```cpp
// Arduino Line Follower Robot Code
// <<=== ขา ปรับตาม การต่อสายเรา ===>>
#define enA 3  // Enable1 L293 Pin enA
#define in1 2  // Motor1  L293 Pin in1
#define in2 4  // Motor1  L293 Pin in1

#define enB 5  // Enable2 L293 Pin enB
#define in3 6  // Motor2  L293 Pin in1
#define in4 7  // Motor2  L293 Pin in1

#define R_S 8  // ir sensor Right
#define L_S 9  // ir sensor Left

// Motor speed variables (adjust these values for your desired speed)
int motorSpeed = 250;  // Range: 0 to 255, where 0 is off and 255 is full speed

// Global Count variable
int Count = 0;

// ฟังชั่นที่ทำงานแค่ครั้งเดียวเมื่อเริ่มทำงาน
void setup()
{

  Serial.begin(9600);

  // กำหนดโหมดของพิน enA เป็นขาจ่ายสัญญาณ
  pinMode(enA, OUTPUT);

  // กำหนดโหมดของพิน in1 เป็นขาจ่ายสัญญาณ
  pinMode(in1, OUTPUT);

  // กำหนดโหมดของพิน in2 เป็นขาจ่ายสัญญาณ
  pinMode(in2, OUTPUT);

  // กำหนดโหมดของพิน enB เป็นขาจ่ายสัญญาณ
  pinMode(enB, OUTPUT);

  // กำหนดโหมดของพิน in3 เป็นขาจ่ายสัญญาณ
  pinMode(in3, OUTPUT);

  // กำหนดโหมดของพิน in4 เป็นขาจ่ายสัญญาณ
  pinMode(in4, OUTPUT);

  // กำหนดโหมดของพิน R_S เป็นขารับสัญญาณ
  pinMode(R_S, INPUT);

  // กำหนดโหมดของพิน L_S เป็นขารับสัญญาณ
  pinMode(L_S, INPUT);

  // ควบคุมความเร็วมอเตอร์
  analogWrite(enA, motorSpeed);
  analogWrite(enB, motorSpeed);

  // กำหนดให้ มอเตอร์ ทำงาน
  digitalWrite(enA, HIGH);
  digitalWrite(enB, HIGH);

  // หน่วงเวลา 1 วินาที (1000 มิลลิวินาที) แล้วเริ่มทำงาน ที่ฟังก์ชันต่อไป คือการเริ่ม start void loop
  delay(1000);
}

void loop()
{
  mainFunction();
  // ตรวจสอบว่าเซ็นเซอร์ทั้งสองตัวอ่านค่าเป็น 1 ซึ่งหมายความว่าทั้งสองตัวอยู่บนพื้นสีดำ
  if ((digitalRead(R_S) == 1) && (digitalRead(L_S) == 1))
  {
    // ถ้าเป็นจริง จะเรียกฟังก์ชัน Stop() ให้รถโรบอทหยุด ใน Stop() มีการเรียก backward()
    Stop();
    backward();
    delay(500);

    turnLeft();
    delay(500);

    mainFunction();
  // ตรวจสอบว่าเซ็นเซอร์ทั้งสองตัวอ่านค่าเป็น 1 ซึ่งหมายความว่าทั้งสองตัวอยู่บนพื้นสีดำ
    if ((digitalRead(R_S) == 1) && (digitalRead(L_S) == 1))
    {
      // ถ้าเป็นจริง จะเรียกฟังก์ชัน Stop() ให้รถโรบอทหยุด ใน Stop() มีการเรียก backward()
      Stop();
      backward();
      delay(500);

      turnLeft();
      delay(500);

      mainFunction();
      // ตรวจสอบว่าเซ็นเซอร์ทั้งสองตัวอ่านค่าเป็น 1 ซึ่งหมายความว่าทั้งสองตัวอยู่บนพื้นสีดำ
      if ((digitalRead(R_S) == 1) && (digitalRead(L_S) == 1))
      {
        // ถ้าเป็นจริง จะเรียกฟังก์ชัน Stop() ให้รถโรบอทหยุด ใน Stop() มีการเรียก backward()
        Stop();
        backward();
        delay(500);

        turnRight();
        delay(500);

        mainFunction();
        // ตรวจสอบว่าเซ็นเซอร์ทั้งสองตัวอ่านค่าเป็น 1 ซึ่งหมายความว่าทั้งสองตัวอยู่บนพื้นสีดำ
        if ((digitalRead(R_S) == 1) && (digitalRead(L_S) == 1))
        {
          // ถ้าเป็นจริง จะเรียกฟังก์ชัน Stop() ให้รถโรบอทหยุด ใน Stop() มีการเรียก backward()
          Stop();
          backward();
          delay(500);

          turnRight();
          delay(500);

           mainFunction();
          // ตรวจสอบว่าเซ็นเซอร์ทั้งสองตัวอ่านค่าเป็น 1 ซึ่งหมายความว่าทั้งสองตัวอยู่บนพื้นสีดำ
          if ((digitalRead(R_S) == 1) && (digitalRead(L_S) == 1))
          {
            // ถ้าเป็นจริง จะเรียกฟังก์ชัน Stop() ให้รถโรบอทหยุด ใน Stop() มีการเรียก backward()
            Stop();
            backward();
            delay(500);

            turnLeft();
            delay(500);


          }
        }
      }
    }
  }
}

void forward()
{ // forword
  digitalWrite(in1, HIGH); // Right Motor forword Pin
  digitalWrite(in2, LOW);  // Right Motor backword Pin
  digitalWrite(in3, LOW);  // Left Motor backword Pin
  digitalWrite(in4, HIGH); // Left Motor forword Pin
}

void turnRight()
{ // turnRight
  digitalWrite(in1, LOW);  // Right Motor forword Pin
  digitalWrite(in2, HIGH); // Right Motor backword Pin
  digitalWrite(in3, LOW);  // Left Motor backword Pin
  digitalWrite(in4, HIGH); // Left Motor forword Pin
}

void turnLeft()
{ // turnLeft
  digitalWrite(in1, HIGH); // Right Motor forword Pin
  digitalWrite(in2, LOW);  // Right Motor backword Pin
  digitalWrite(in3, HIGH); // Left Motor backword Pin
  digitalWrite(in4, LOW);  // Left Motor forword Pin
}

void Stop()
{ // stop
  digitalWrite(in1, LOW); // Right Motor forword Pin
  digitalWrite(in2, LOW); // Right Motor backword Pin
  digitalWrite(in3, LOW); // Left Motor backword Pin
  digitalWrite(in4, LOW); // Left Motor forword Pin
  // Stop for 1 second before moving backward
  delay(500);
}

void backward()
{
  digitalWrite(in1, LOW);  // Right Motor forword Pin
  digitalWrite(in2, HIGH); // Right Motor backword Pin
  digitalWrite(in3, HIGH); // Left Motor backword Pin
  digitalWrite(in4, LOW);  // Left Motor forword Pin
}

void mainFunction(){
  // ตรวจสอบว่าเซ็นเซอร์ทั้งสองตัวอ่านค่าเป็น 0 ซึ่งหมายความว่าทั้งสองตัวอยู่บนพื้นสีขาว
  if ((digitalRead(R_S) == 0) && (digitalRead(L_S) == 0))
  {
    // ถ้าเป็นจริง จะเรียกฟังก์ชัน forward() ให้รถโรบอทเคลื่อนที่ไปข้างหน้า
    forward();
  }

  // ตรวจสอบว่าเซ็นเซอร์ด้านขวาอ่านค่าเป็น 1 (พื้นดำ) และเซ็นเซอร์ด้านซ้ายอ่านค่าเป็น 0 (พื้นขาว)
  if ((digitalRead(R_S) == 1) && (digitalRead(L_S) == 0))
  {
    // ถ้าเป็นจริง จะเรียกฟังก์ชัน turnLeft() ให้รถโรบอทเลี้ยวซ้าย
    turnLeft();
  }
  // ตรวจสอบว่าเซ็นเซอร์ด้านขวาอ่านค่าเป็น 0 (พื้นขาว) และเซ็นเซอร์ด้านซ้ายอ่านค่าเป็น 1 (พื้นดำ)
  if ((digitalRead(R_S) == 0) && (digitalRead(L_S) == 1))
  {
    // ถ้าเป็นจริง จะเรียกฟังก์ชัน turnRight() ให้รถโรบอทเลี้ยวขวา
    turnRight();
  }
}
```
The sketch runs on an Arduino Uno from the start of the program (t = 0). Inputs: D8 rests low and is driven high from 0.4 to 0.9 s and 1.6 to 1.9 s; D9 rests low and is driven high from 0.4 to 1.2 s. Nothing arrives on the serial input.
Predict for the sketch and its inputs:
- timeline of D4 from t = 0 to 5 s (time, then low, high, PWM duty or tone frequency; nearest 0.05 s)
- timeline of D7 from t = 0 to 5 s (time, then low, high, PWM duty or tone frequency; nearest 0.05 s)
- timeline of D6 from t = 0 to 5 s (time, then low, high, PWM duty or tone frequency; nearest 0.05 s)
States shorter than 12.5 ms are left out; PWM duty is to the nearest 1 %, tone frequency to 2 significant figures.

0 s low; 1 s high; 1.2 s low
0 s low; 1 s high; 1.6 s low; 1.9 s high
0 s low; 1.6 s high; 1.9 s low
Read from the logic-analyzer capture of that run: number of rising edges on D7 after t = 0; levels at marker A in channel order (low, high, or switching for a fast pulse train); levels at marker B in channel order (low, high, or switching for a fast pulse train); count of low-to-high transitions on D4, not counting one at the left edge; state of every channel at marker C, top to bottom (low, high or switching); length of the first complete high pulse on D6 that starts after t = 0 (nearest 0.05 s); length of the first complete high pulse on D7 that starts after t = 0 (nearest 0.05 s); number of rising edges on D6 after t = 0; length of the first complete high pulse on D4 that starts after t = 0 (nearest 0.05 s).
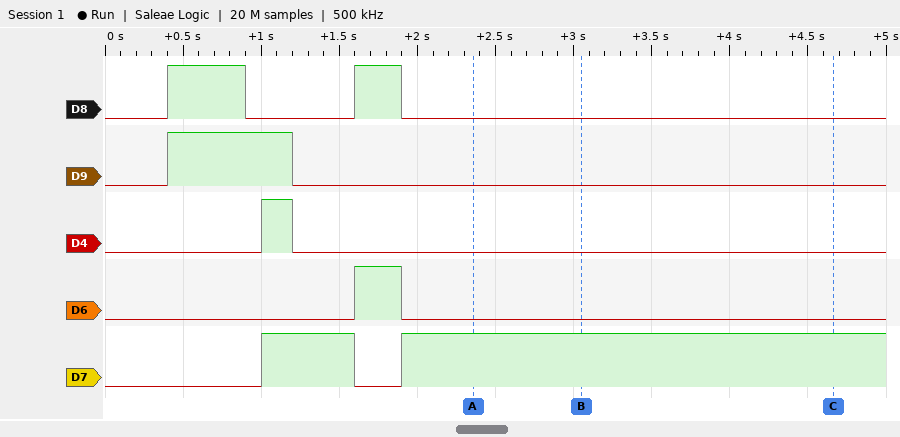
2
D8 low, D9 low, D4 low, D6 low, D7 high
D8 low, D9 low, D4 low, D6 low, D7 high
1
D8 low, D9 low, D4 low, D6 low, D7 high
0.30 s
0.60 s
1
0.20 s
